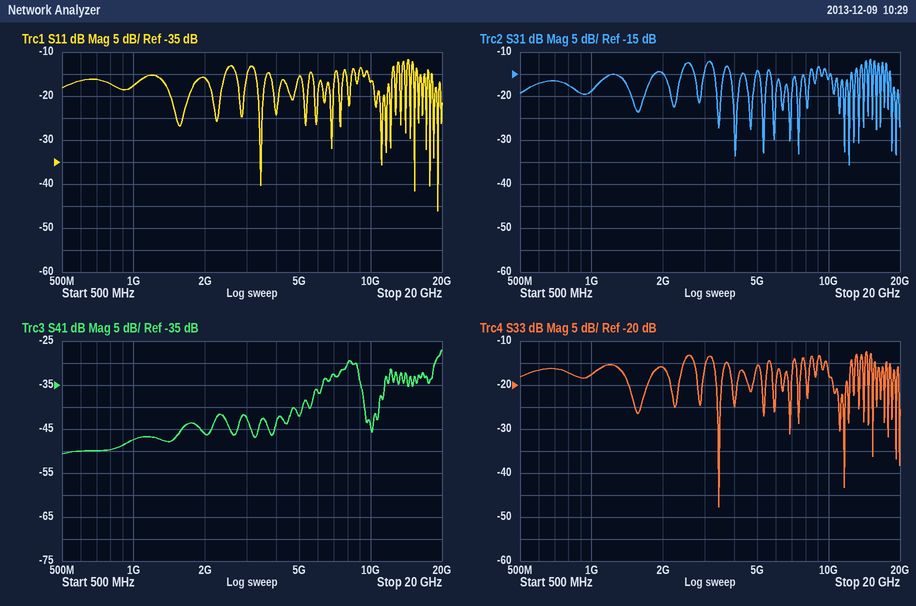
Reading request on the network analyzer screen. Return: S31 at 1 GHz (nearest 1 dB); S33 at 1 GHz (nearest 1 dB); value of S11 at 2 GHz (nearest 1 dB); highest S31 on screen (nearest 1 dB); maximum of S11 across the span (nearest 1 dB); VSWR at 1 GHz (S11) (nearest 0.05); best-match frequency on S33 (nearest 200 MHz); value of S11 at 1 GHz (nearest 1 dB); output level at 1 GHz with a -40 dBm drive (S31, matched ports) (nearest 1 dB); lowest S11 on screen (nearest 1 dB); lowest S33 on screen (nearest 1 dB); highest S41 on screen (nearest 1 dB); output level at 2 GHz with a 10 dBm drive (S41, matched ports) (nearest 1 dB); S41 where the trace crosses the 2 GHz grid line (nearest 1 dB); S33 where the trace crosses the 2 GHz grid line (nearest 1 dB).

-19 dB
-18 dB
-16 dB
-12 dB
-12 dB
1.30
3.4 GHz
-18 dB
-59 dBm
-46 dB
-48 dB
-27 dB
-36 dBm
-46 dB
-16 dB
